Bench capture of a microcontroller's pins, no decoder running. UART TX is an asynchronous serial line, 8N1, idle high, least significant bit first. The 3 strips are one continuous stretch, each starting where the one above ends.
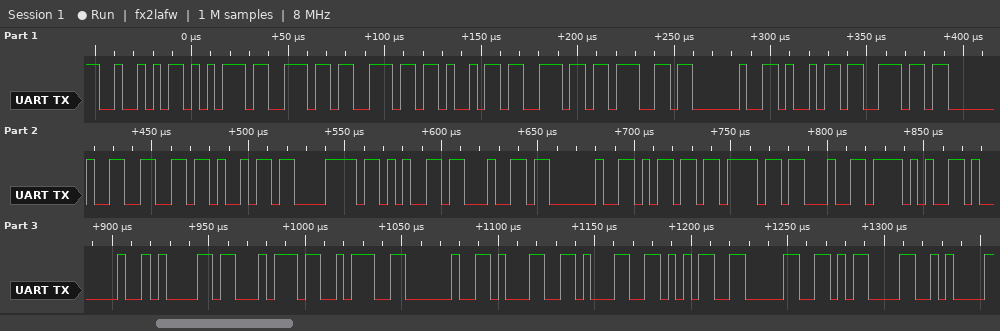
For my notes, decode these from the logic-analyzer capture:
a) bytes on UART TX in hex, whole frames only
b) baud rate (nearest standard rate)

52 75 6E 6E 69 6E 67 20 69 6E 20 66 69 78 65 64 20 6D 6F 64 65 20 61 74 3A 20 31 31 35 30 0D 0A
250000 baud
